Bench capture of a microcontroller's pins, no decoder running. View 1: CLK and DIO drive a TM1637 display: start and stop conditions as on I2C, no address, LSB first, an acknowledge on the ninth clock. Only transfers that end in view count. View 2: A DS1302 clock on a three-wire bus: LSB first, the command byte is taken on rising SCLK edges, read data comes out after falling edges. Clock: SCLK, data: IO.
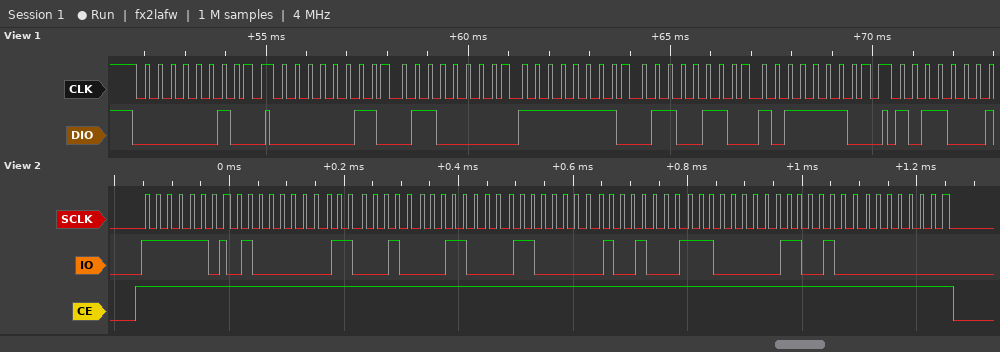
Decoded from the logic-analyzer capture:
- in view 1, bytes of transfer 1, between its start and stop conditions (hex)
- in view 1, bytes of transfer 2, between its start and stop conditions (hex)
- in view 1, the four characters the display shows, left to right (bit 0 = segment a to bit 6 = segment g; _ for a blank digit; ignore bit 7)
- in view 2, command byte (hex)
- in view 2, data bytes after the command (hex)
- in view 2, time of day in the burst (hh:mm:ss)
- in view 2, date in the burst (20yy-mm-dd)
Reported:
40
C0 06 FF 66 7D
1846
0xBF
02 46 18 06 12 07 26 00
18:46:02
2026-12-06
